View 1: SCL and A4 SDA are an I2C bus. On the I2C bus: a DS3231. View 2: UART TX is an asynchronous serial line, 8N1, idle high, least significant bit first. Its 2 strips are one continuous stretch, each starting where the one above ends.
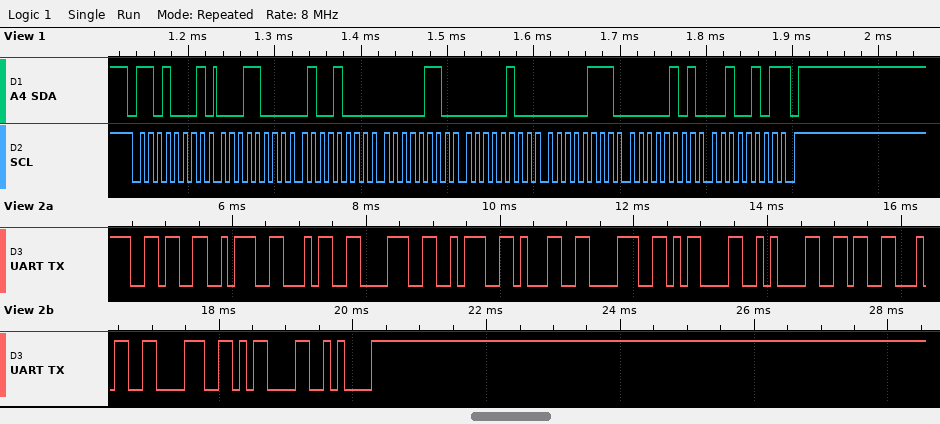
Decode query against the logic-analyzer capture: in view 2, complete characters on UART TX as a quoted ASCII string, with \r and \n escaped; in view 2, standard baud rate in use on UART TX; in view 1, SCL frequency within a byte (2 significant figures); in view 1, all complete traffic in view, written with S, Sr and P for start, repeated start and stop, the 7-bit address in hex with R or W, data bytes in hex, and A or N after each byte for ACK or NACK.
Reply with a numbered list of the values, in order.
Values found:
1. "6:48:18\r\n648\r\n"
2. 9600 baud
3. 100 kHz
4. S 68R A 18 A 48 A 06 A 04 A 07 A 05 A 25 N P
